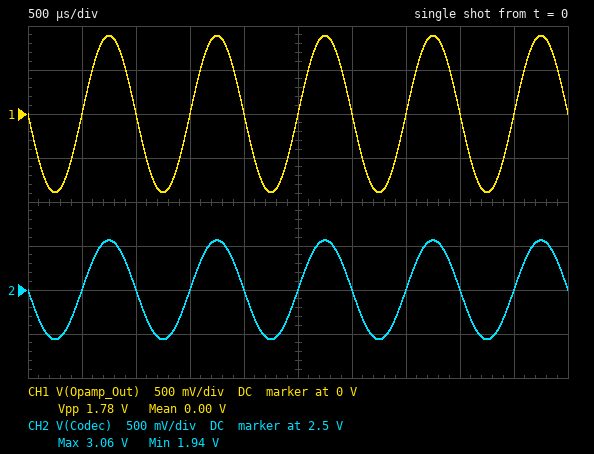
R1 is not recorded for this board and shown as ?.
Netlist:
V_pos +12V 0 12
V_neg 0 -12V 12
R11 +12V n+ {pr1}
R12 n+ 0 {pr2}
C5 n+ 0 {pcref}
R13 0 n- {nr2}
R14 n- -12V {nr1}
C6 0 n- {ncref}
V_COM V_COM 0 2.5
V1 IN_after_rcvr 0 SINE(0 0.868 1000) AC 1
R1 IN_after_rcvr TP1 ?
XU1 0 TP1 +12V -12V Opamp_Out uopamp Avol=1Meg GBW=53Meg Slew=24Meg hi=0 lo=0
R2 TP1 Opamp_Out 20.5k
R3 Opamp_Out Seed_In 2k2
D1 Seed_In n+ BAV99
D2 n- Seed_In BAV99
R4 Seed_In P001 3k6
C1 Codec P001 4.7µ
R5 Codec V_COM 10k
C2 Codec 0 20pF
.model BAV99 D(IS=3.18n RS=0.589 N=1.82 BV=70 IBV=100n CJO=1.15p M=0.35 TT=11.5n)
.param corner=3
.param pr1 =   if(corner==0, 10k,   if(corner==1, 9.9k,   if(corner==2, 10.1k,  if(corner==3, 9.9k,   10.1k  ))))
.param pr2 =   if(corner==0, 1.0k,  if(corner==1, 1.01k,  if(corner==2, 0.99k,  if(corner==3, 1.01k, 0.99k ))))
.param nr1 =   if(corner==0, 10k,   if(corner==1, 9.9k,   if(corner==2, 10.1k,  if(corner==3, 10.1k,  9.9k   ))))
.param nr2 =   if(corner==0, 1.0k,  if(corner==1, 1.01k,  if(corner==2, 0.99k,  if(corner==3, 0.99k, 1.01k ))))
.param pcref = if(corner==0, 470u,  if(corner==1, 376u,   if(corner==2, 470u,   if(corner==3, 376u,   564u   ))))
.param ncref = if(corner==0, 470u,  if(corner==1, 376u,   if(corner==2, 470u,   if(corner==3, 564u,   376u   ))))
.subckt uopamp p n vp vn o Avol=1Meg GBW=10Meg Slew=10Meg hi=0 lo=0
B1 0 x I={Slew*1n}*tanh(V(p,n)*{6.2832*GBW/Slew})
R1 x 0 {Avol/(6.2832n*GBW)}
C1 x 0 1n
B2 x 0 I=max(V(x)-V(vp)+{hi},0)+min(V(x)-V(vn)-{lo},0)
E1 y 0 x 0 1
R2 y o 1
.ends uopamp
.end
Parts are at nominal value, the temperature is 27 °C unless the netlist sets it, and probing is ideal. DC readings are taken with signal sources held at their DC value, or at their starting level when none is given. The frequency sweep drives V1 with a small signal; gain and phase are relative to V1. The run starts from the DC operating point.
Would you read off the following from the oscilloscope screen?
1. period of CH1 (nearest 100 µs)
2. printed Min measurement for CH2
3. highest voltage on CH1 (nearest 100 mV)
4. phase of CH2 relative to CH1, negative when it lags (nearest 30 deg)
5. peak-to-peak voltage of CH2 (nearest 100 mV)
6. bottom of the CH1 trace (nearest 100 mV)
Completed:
1.0 ms
1.94 V
900 mV
0 deg
1.1 V
-900 mV
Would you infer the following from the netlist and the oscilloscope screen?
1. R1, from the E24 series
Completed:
20 kΩ
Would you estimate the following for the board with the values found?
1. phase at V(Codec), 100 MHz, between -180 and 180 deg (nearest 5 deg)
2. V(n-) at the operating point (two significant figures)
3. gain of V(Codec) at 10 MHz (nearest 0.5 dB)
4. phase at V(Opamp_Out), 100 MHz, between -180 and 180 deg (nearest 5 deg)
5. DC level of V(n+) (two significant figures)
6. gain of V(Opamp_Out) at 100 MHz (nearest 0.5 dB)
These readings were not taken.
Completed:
-40 deg
-1.1 V
-18.0 dB
105 deg
1.1 V
-11.5 dB
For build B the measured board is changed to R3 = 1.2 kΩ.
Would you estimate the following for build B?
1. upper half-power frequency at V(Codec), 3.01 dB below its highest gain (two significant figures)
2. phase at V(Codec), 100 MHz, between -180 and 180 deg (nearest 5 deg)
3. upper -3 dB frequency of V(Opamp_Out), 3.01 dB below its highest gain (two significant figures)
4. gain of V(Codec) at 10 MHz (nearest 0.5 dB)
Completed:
2.4 MHz
-30 deg
26 MHz
-16.5 dB
